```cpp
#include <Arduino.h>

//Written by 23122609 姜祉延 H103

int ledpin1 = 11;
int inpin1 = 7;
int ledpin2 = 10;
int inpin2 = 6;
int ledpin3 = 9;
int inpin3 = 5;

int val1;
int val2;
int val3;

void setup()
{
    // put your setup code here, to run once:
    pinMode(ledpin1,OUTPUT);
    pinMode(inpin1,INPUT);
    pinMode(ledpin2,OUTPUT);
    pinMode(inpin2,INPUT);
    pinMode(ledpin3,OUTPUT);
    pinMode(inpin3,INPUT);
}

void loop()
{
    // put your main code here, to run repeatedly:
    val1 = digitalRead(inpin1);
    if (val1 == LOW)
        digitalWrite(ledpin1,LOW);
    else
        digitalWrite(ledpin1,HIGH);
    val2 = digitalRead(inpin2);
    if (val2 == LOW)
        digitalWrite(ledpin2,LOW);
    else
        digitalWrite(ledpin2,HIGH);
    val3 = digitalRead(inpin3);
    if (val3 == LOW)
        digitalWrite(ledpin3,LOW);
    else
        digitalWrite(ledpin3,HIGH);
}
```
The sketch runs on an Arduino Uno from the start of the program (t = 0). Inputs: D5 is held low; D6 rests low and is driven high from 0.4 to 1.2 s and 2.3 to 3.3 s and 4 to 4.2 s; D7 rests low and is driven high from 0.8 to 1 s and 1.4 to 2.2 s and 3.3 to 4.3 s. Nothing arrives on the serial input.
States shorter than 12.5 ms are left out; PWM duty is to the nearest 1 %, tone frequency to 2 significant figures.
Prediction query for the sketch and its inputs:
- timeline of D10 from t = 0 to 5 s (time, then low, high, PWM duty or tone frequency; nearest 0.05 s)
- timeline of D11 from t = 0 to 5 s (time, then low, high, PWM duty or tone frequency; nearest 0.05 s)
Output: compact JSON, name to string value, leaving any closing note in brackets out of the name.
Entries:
{"timeline of D10 from t = 0 to 5 s": "0 s low; 0.4 s high; 1.2 s low; 2.3 s high; 3.3 s low; 4 s high; 4.2 s low", "timeline of D11 from t = 0 to 5 s": "0 s low; 0.8 s high; 1 s low; 1.4 s high; 2.2 s low; 3.3 s high; 4.3 s low"}
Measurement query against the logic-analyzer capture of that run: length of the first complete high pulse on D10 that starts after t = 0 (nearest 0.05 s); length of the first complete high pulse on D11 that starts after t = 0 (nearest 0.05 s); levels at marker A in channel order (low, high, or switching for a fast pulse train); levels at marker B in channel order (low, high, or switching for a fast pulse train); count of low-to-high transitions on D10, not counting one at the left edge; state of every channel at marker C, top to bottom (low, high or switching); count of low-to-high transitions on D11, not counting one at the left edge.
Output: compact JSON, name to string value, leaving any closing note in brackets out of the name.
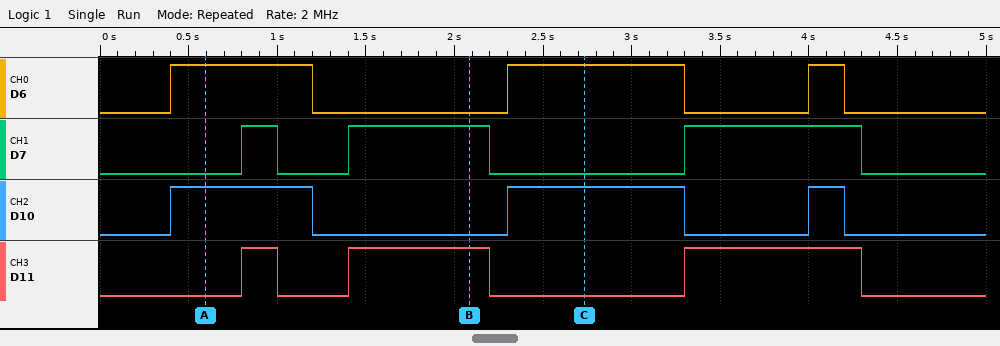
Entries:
{"length of the first complete high pulse on D10 that starts after t = 0": "0.80 s", "length of the first complete high pulse on D11 that starts after t = 0": "0.20 s", "levels at marker A in channel order": "D6 high, D7 low, D10 high, D11 low", "levels at marker B in channel order": "D6 low, D7 high, D10 low, D11 high", "count of low-to-high transitions on D10, not counting one at the left edge": "3", "state of every channel at marker C, top to bottom": "D6 high, D7 low, D10 high, D11 low", "count of low-to-high transitions on D11, not counting one at the left edge": "3"}
